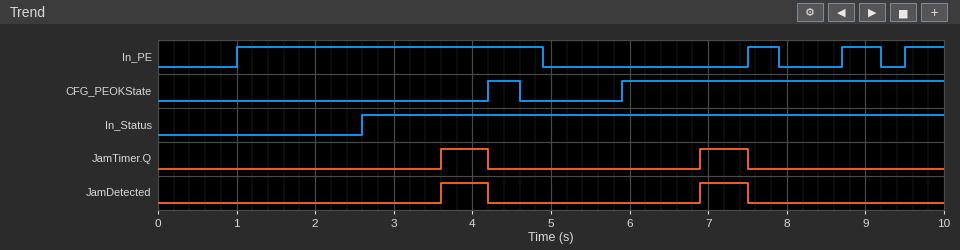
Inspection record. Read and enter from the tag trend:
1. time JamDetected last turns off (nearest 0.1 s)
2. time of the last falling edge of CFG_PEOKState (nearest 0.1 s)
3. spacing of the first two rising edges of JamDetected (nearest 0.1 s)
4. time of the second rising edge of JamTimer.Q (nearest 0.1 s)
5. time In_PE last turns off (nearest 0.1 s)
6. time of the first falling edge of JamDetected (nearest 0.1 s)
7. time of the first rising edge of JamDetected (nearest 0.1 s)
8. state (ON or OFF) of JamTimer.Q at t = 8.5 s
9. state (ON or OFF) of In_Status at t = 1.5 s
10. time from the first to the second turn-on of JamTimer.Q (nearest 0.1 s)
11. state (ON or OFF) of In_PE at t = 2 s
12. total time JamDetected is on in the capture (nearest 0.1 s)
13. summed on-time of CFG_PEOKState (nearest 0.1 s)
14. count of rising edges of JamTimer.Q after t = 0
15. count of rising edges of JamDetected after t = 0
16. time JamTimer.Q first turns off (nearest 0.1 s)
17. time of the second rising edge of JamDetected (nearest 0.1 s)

7.5 s
4.6 s
3.3 s
6.9 s
9.2 s
4.2 s
3.6 s
OFF
OFF
3.3 s
ON
1.2 s
4.5 s
2
2
4.2 s
6.9 s
